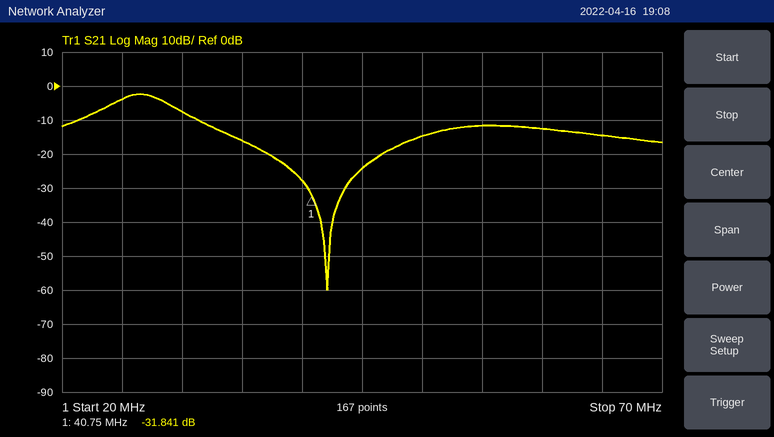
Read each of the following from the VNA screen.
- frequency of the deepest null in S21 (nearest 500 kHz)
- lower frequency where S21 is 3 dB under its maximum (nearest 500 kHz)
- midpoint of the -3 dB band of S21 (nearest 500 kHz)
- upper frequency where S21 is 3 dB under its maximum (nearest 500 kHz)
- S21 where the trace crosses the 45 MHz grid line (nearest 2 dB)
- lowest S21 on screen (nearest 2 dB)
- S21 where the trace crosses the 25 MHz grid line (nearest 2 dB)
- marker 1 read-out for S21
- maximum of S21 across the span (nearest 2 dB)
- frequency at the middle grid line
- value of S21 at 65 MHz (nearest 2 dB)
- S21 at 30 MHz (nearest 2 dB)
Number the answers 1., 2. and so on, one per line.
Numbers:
1. 42.0 MHz
2. 24.0 MHz
3. 26.5 MHz
4. 29.0 MHz
5. -24 dB
6. -60 dB
7. -4 dB
8. -31.841 dB
9. -2 dB
10. 45 MHz
11. -14 dB
12. -8 dB
